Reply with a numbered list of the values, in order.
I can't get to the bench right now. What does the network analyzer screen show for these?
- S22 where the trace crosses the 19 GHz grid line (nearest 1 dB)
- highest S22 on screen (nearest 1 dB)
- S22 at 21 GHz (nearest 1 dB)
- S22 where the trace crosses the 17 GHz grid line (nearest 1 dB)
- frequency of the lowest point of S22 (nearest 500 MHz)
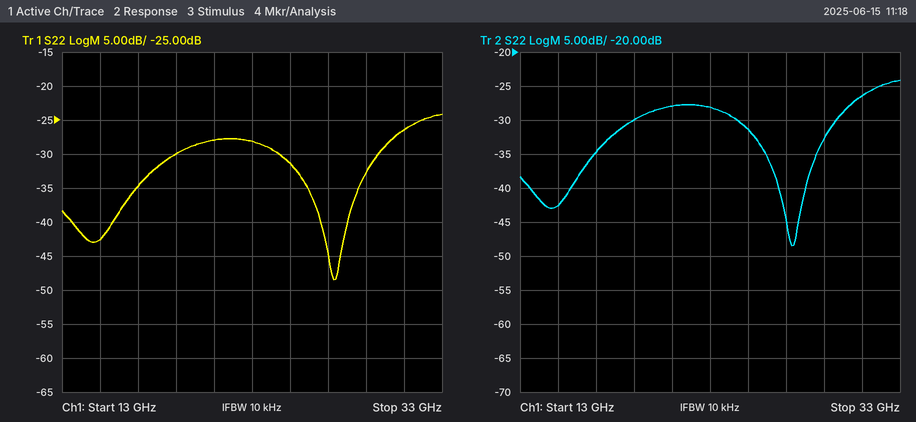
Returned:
1. -30 dB
2. -24 dB
3. -28 dB
4. -35 dB
5. 27.5 GHz
